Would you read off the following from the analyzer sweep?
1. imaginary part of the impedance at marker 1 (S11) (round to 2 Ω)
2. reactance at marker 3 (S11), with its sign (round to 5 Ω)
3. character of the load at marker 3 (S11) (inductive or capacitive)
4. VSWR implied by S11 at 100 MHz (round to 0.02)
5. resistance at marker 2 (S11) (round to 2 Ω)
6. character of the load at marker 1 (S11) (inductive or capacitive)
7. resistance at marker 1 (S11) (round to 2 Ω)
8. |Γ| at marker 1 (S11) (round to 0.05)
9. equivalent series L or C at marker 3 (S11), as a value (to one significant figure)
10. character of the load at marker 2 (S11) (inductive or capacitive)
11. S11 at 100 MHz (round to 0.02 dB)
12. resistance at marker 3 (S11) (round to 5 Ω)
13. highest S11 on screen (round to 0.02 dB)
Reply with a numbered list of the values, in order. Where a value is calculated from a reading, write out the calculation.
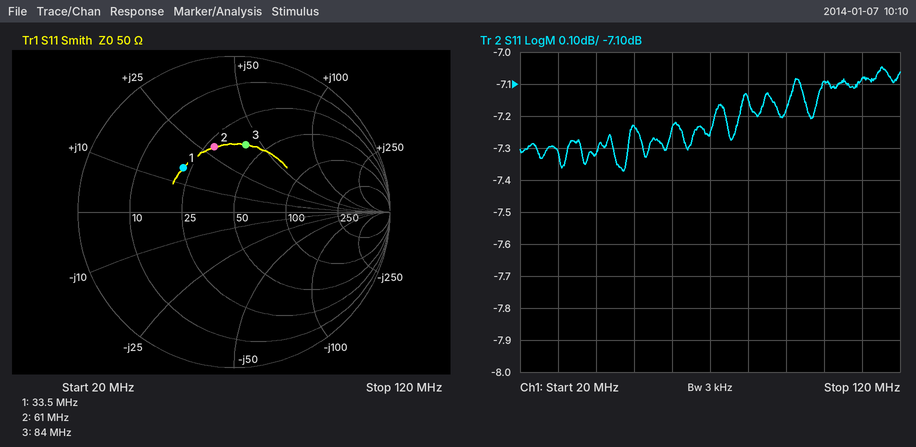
1. +16 Ω
2. +40 Ω
3. inductive
4. |Γ| = 10^(-7.1/20) = 0.4416; VSWR = (1 + 0.4416)/(1 − 0.4416) ≈ 2.58
5. 28 Ω
6. inductive
7. 22 Ω
8. 0.45
9. L = 40 Ω/(2π × 84 MHz) ≈ 75.8 nH, so 80 nH to one significant figure
10. inductive
11. -7.10 dB
12. 40 Ω
13. -7.04 dB
